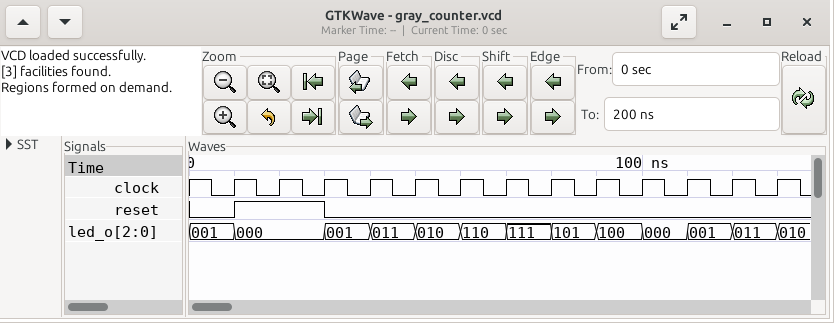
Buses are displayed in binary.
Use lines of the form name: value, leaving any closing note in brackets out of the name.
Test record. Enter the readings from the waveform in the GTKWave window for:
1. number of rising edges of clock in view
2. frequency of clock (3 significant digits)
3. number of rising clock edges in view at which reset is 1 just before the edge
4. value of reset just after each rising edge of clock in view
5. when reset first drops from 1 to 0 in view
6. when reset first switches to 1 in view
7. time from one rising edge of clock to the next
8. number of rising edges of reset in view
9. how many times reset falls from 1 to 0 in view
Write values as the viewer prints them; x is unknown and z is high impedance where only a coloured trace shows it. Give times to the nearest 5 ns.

number of rising edges of clock in view: 13
frequency of clock: 100 MHz
number of rising clock edges in view at which reset is 1 just before the edge: 2
value of reset just after each rising edge of clock in view: 1 1 0 0 0 0 0 0 0 0 0 0 0
when reset first drops from 1 to 0 in view: 30 ns
when reset first switches to 1 in view: 10 ns
time from one rising edge of clock to the next: 10 ns
number of rising edges of reset in view: 1
how many times reset falls from 1 to 0 in view: 1
